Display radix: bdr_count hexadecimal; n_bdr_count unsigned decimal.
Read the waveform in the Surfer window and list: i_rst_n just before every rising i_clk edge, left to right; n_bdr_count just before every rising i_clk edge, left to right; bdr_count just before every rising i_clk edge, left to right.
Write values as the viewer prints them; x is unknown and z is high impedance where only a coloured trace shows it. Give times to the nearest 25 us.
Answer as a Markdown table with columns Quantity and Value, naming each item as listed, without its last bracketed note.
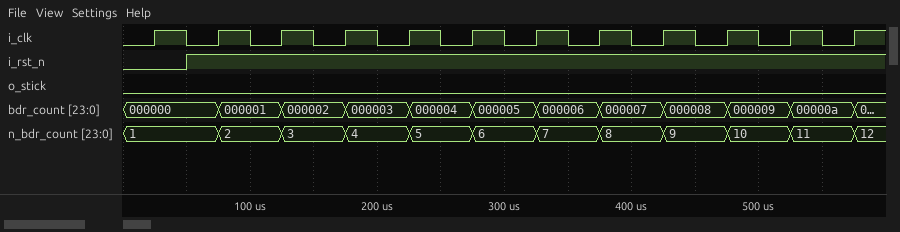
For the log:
| Quantity | Value |
|---|---|
| i_rst_n just before every rising i_clk edge, left to right | 0 1 1 1 1 1 1 1 1 1 1 1 |
| n_bdr_count just before every rising i_clk edge, left to right | 1, 1, 2, 3, 4, 5, 6, 7, 8, 9, 10, 11 |
| bdr_count just before every rising i_clk edge, left to right | 000000, 000000, 000001, 000002, 000003, 000004, 000005, 000006, 000007, 000008, 000009, 00000a |
